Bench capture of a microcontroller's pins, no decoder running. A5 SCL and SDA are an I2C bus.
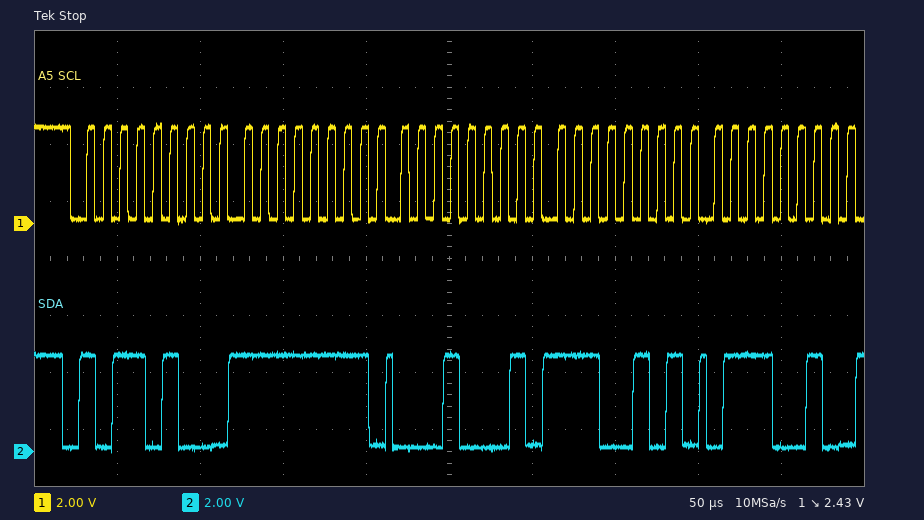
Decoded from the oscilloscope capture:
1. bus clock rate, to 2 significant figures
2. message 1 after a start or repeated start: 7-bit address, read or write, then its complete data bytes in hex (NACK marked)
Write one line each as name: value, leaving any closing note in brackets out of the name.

bus clock rate, to 2 significant figures: 100 kHz
message 1 after a start or repeated start: 7-bit address, read or write, then its complete data bytes in hex: 0x5A write: FF 11 E5 72
